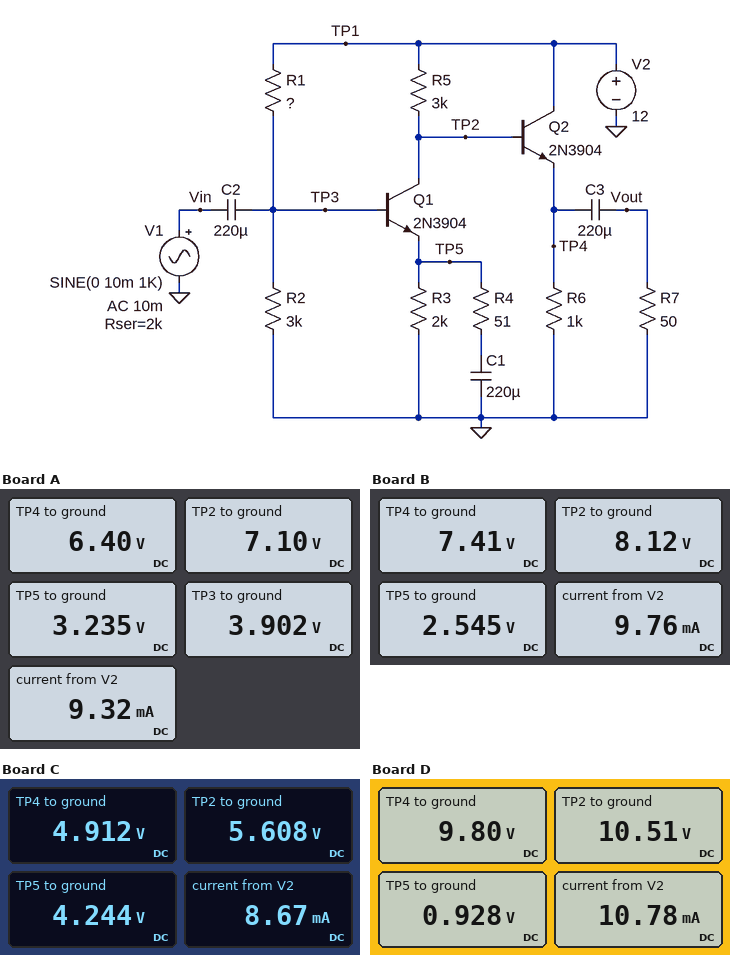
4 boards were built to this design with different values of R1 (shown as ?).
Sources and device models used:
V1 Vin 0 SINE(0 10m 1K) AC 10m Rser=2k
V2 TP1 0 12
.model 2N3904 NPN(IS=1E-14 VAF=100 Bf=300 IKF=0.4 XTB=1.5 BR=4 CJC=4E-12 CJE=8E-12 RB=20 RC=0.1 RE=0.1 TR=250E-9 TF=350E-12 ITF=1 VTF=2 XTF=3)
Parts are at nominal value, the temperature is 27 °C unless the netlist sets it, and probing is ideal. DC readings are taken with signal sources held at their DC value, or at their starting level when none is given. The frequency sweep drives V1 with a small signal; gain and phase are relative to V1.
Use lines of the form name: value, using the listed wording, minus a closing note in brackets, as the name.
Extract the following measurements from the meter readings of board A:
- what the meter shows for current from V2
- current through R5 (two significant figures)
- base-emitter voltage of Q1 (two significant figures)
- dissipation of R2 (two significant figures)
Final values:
what the meter shows for current from V2: 9.32 mA
current through R5: 1.6 mA
base-emitter voltage of Q1: 670 mV
dissipation of R2: 5.1 mW
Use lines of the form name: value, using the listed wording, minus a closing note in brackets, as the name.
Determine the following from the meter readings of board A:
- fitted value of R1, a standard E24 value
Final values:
fitted value of R1, a standard E24 value: 6.2 kΩ
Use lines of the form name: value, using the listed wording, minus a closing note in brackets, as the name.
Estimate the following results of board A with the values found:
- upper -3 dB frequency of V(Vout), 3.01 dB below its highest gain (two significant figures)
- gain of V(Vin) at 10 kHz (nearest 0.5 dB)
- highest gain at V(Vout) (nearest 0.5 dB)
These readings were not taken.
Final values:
upper -3 dB frequency of V(Vout), 3.01 dB below its highest gain: 1.3 MHz
gain of V(Vin) at 10 kHz: -6.5 dB
highest gain at V(Vout): 24.5 dB
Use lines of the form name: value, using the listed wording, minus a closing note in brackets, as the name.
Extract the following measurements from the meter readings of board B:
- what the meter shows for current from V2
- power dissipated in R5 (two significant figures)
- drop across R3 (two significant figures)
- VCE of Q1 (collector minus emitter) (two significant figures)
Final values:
what the meter shows for current from V2: 9.76 mA
power dissipated in R5: 5.0 mW
drop across R3: 2.5 V
VCE of Q1 (collector minus emitter): 5.6 V
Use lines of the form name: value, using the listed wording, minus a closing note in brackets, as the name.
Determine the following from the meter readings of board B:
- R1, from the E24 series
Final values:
R1, from the E24 series: 8.2 kΩ
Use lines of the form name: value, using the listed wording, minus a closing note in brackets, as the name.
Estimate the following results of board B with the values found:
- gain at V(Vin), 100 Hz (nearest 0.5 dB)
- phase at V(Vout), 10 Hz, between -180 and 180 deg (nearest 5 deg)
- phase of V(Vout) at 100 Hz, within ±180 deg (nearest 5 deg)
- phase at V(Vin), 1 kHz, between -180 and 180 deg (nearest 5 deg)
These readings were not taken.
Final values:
gain at V(Vin), 100 Hz: -6.0 dB
phase at V(Vout), 10 Hz, between -180 and 180 deg: -90 deg
phase of V(Vout) at 100 Hz, within ±180 deg: -170 deg
phase at V(Vin), 1 kHz, between -180 and 180 deg: 0 deg
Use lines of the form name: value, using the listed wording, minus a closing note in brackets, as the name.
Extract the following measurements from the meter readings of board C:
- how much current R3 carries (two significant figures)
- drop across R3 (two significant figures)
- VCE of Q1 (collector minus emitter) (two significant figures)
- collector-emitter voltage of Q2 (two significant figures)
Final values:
how much current R3 carries: 2.1 mA
drop across R3: 4.2 V
VCE of Q1 (collector minus emitter): 1.4 V
collector-emitter voltage of Q2: 7.1 V
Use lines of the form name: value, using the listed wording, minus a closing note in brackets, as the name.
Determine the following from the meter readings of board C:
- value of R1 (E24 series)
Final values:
value of R1: 4.3 kΩ
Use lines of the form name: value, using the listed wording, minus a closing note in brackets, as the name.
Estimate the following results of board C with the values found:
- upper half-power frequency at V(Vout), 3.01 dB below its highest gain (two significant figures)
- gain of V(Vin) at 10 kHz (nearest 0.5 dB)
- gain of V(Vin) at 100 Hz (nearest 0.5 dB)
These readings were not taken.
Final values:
upper half-power frequency at V(Vout), 3.01 dB below its highest gain: 1.0 MHz
gain of V(Vin) at 10 kHz: -7.0 dB
gain of V(Vin) at 100 Hz: -7.0 dB
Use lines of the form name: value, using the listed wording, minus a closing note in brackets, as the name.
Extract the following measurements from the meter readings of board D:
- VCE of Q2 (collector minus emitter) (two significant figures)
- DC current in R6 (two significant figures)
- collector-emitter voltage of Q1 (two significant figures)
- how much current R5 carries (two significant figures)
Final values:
VCE of Q2 (collector minus emitter): 2.2 V
DC current in R6: 9.8 mA
collector-emitter voltage of Q1: 9.6 V
how much current R5 carries: 500 µA
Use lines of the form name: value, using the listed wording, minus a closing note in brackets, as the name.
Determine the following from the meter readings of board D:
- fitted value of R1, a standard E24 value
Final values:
fitted value of R1, a standard E24 value: 20 kΩ
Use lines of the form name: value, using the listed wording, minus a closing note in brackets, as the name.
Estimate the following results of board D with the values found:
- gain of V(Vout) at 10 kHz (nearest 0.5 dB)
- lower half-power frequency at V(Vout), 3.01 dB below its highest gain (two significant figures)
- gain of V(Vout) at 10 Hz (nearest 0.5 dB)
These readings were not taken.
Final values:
gain of V(Vout) at 10 kHz: 21.5 dB
lower half-power frequency at V(Vout), 3.01 dB below its highest gain: 14 Hz
gain of V(Vout) at 10 Hz: 16.5 dB
